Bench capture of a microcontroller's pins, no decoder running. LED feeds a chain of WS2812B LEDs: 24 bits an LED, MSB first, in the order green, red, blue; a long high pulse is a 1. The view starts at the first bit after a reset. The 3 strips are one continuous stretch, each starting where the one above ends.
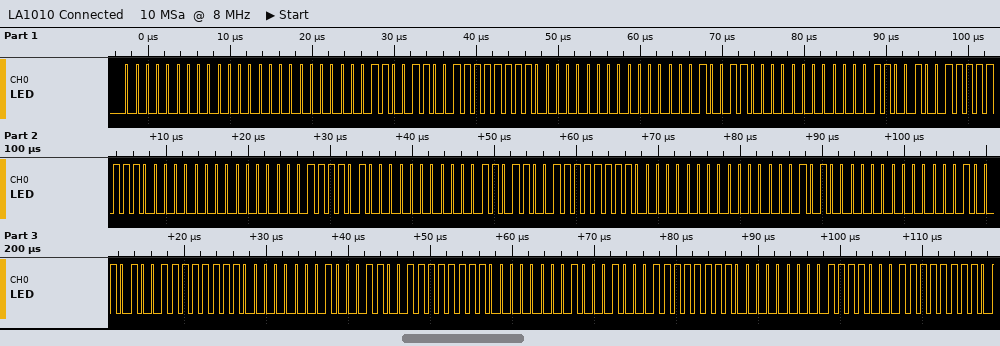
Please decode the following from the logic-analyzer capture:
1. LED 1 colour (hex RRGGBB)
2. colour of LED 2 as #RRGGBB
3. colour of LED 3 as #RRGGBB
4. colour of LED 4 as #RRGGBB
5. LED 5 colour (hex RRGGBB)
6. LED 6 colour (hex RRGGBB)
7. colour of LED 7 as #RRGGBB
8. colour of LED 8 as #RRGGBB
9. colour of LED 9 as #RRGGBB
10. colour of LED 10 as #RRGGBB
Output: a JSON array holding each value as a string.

["#000000", "#FFCC00", "#980000", "#FF6400", "#F40000", "#FF6C00", "#A00000", "#FF9400", "#FF8C00", "#FF8800"]
